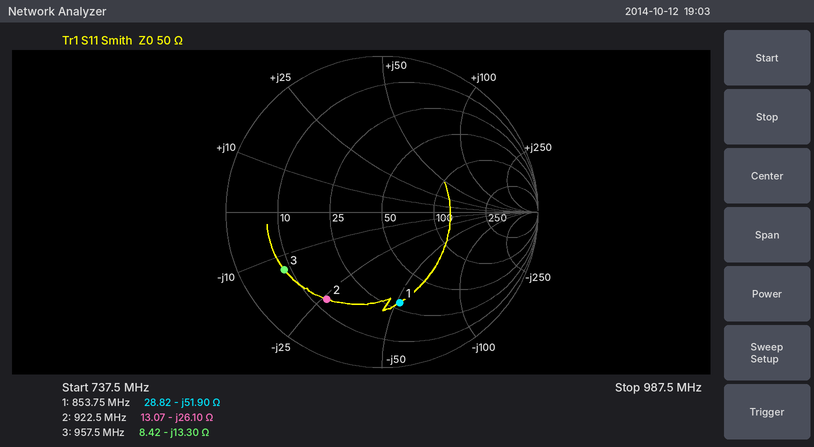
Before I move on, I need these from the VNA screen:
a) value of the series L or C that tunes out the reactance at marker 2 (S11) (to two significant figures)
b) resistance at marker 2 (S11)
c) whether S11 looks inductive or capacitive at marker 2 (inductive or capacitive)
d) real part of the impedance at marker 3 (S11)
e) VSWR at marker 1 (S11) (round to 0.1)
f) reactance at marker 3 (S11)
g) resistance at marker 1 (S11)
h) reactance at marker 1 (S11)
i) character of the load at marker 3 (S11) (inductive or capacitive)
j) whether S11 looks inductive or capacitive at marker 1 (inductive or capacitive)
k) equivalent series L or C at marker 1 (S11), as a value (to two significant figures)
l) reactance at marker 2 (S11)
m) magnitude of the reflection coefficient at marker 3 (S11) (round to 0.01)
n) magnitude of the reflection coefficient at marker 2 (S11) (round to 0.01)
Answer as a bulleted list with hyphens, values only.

- 4.5 nH
- 13.07 Ω
- capacitive
- 8.42 Ω
- 3.9
- -13.30 Ω
- 28.82 Ω
- -51.90 Ω
- capacitive
- capacitive
- 3.6 pF
- -26.10 Ω
- 0.73
- 0.66
